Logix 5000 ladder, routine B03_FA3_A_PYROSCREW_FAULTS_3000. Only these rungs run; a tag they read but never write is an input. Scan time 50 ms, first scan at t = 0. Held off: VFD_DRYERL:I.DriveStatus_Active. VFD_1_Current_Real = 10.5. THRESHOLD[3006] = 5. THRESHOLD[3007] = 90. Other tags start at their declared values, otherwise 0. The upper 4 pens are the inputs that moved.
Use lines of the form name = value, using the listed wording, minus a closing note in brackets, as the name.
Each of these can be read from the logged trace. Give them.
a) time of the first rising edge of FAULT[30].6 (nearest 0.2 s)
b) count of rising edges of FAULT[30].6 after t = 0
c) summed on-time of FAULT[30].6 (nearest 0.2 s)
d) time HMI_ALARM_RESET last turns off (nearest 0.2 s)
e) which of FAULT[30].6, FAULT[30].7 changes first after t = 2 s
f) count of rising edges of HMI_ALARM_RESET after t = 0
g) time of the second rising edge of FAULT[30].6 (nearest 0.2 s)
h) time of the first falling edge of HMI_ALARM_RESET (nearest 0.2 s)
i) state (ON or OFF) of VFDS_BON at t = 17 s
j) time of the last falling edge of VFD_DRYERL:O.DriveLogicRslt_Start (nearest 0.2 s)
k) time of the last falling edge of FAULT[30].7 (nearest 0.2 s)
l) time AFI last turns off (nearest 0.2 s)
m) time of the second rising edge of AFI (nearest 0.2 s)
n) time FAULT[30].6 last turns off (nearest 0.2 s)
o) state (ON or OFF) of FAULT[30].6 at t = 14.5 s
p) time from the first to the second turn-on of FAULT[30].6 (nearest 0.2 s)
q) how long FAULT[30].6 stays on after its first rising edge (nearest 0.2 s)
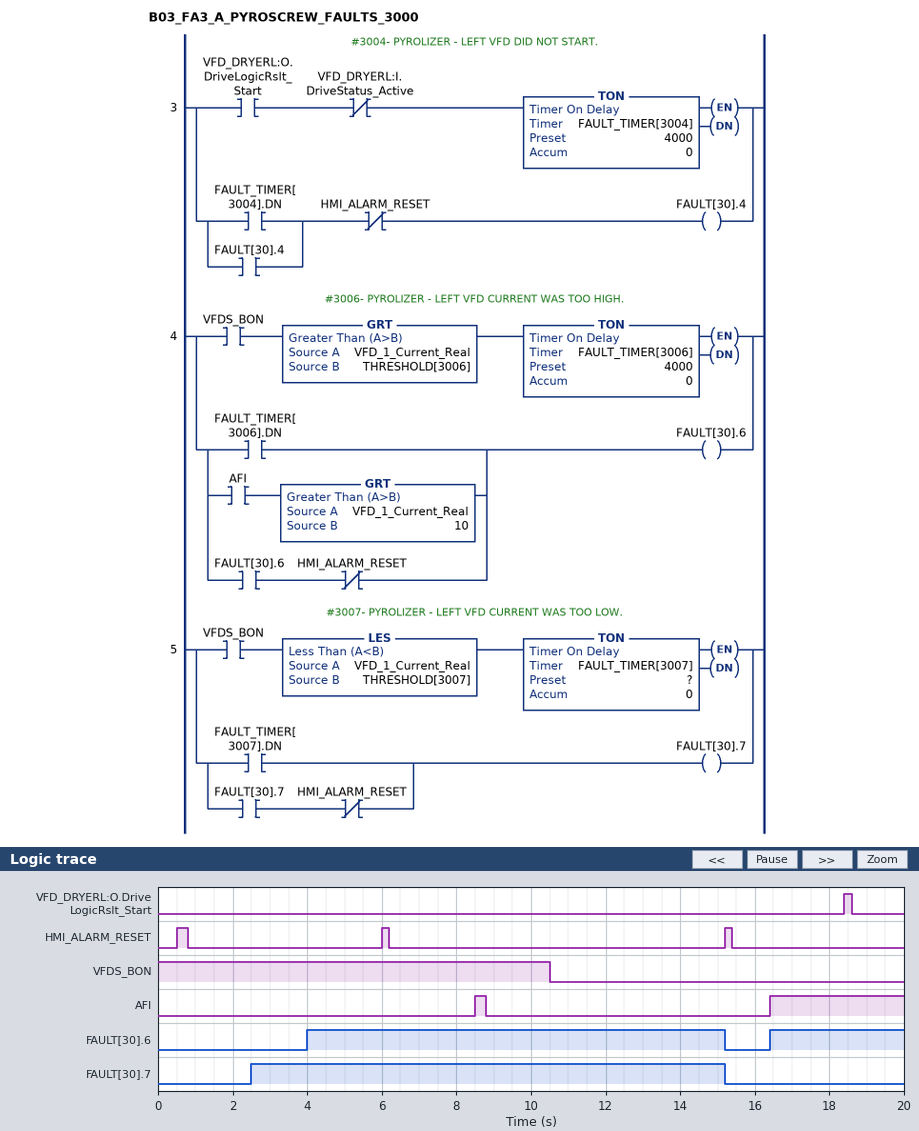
time of the first rising edge of FAULT[30].6 = 4.0 s
count of rising edges of FAULT[30].6 after t = 0 = 2
summed on-time of FAULT[30].6 = 14.8 s
time HMI_ALARM_RESET last turns off = 15.4 s
which of FAULT[30].6, FAULT[30].7 changes first after t = 2 s = FAULT[30].7
count of rising edges of HMI_ALARM_RESET after t = 0 = 3
time of the second rising edge of FAULT[30].6 = 16.4 s
time of the first falling edge of HMI_ALARM_RESET = 0.8 s
state (ON or OFF) of VFDS_BON at t = 17 s = OFF
time of the last falling edge of VFD_DRYERL:O.DriveLogicRslt_Start = 18.6 s
time of the last falling edge of FAULT[30].7 = 15.2 s
time AFI last turns off = 8.8 s
time of the second rising edge of AFI = 16.4 s
time FAULT[30].6 last turns off = 15.2 s
state (ON or OFF) of FAULT[30].6 at t = 14.5 s = ON
time from the first to the second turn-on of FAULT[30].6 = 12.4 s
how long FAULT[30].6 stays on after its first rising edge = 11.2 s
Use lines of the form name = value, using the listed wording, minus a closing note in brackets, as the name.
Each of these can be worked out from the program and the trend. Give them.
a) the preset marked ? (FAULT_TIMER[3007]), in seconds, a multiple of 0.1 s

the preset marked ? (FAULT_TIMER[3007]), in seconds, a multiple of 0.1 s = 2.5 s
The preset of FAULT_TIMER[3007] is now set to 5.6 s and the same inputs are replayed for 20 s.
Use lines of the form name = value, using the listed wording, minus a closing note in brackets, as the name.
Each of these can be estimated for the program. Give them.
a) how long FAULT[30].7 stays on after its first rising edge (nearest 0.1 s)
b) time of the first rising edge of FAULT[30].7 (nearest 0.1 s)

how long FAULT[30].7 stays on after its first rising edge = 9.6 s
time of the first rising edge of FAULT[30].7 = 5.6 s
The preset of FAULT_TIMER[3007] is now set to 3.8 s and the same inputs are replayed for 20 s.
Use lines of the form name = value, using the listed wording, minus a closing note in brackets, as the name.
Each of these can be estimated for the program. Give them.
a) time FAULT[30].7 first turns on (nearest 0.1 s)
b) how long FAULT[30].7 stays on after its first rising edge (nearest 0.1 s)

time FAULT[30].7 first turns on = 3.8 s
how long FAULT[30].7 stays on after its first rising edge = 11.4 s
